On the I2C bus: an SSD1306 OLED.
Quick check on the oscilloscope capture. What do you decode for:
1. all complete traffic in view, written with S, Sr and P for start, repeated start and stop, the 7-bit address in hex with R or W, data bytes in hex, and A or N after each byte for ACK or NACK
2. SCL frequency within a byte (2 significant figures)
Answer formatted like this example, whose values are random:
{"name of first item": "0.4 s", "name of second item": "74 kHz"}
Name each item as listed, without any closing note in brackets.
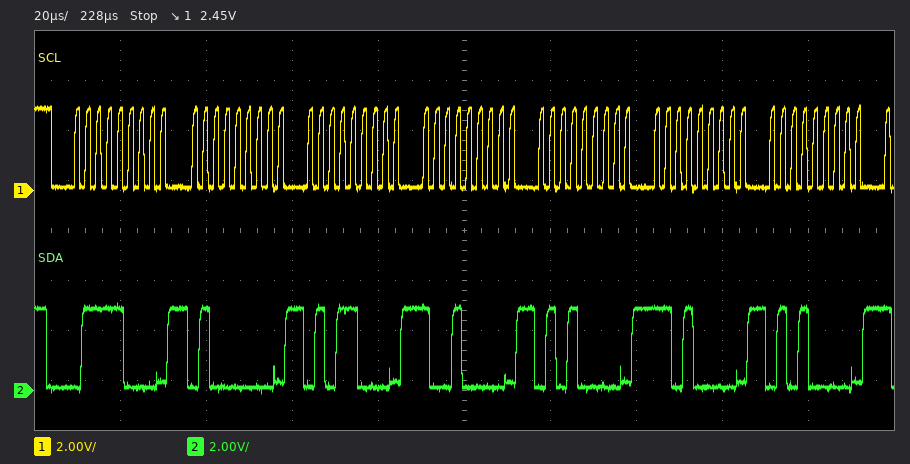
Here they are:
{"all complete traffic in view, written with S, Sr and P for start, repeated start and stop, the 7-bit address in hex with R or W, data bytes in hex, and A or N after each byte for ACK or NACK": "S 3CW A 40 A 58 A 90 A 50 A D0 A 50 A", "SCL frequency within a byte": "400 kHz"}
